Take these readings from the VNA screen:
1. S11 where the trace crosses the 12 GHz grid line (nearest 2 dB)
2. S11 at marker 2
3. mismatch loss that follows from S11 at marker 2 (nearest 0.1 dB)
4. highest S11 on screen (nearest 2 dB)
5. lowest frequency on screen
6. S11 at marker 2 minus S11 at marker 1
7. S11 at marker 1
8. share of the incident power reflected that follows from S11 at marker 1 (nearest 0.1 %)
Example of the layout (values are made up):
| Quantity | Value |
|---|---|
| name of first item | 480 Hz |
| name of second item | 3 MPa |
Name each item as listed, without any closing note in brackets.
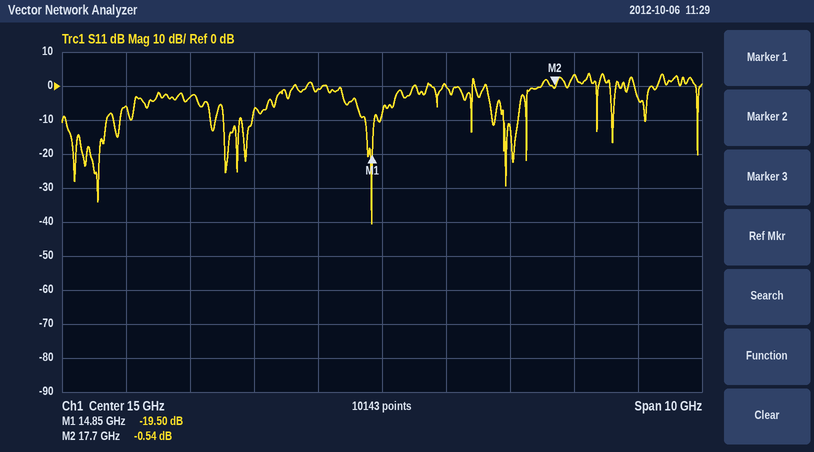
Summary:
| Quantity | Value |
|---|---|
| S11 where the trace crosses the 12 GHz grid line | -4 dB |
| S11 at marker 2 | -0.54 dB |
| mismatch loss that follows from S11 at marker 2 | 9.3 dB |
| highest S11 on screen | 4 dB |
| lowest frequency on screen | 10 GHz |
| S11 at marker 2 minus S11 at marker 1 | 18.96 dB |
| S11 at marker 1 | -19.50 dB |
| share of the incident power reflected that follows from S11 at marker 1 | 1.1 % |
